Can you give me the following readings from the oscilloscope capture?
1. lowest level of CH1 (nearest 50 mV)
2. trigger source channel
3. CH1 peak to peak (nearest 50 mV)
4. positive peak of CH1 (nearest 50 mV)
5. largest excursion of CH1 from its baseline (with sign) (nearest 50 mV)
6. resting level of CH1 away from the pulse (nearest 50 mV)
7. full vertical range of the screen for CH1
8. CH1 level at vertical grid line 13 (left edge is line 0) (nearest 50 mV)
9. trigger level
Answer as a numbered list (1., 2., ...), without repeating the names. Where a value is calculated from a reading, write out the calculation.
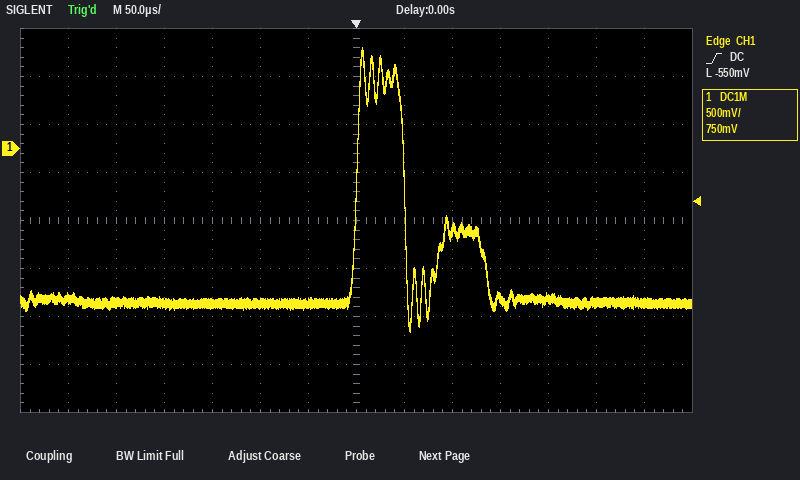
1. -1.90 V
2. CH1
3. 1.05 V − (-1.90 V) = 2.95 V
4. 1.05 V
5. 1.05 V − (-1.60 V) = +2.65 V
6. -1.60 V
7. 4 V
8. -1.60 V
9. -550 mV
